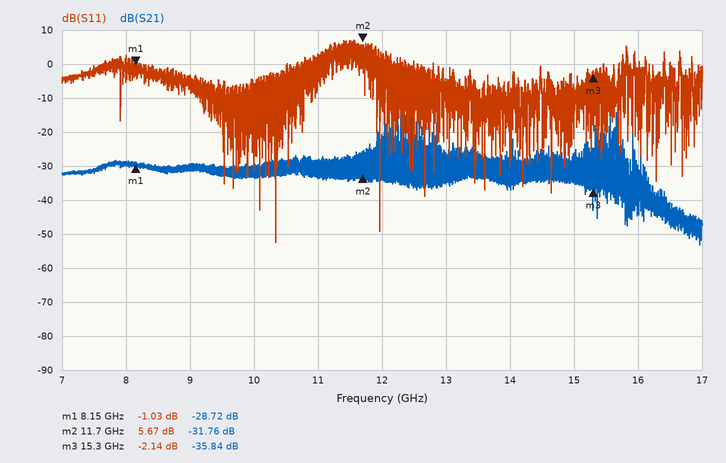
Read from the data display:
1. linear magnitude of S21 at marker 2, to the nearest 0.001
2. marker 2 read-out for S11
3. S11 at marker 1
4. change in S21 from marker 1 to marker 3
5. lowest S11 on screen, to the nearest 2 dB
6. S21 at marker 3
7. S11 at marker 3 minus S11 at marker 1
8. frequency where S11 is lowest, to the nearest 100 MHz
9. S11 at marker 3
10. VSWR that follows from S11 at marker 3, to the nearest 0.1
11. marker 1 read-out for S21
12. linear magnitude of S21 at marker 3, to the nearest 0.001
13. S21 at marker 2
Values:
0.026
5.67 dB
-1.03 dB
-7.12 dB
-52 dB
-35.84 dB
-1.11 dB
10.3 GHz
-2.14 dB
8.2
-28.72 dB
0.016
-31.76 dB
